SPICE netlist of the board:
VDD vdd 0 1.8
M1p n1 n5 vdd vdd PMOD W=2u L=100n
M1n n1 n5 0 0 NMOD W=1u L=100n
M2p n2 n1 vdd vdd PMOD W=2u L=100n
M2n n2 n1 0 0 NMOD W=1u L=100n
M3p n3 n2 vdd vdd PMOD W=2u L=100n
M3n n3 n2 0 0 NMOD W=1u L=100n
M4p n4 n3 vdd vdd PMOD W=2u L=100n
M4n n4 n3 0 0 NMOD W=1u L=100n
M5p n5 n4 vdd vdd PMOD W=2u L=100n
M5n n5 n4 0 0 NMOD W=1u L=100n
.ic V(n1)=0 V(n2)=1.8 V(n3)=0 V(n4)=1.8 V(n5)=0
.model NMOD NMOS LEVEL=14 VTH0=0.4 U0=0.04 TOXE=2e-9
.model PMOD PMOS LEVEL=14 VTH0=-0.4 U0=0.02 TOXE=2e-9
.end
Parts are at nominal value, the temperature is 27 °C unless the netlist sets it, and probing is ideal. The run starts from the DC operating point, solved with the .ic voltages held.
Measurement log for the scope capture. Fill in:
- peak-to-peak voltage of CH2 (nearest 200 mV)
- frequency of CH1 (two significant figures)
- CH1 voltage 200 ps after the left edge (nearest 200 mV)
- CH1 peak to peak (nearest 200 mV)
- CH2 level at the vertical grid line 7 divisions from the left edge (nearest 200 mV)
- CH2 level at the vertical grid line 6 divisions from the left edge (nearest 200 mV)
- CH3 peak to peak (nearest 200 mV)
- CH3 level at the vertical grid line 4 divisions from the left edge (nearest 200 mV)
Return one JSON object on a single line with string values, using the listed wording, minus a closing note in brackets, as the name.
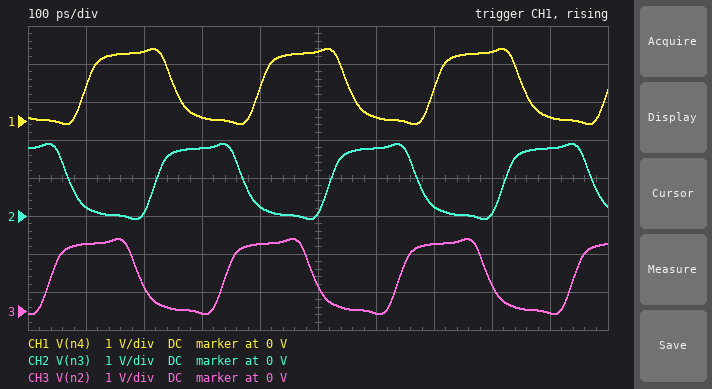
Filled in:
{"peak-to-peak voltage of CH2": "2.0 V", "frequency of CH1": "3.3 GHz", "CH1 voltage 200 ps after the left edge": "1.8 V", "CH1 peak to peak": "2.0 V", "CH2 level at the vertical grid line 7 divisions from the left edge": "200 mV", "CH2 level at the vertical grid line 6 divisions from the left edge": "1.8 V", "CH3 peak to peak": "2.0 V", "CH3 level at the vertical grid line 4 divisions from the left edge": "1.8 V"}
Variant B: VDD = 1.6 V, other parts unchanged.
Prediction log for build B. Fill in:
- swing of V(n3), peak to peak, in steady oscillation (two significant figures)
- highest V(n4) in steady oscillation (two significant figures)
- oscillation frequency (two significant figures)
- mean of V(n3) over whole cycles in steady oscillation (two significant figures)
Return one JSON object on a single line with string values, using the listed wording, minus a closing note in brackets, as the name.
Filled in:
{"swing of V(n3), peak to peak, in steady oscillation": "1.8 V", "highest V(n4) in steady oscillation": "1.7 V", "oscillation frequency": "2.9 GHz", "mean of V(n3) over whole cycles in steady oscillation": "820 mV"}
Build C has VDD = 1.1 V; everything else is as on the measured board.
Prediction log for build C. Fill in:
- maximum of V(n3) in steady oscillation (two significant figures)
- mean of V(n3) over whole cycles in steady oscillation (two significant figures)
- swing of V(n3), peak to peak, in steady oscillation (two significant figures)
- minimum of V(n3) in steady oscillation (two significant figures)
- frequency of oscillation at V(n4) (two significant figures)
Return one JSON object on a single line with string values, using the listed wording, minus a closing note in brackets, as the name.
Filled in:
{"maximum of V(n3) in steady oscillation": "1.2 V", "mean of V(n3) over whole cycles in steady oscillation": "560 mV", "swing of V(n3), peak to peak, in steady oscillation": "1.3 V", "minimum of V(n3) in steady oscillation": "-110 mV", "frequency of oscillation at V(n4)": "1.5 GHz"}
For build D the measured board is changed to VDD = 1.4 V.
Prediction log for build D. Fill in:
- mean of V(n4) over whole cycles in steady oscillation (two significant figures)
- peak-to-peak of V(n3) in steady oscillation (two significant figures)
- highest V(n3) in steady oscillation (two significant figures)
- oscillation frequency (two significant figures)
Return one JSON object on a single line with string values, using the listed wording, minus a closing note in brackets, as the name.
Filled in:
{"mean of V(n4) over whole cycles in steady oscillation": "710 mV", "peak-to-peak of V(n3) in steady oscillation": "1.6 V", "highest V(n3) in steady oscillation": "1.5 V", "oscillation frequency": "2.4 GHz"}
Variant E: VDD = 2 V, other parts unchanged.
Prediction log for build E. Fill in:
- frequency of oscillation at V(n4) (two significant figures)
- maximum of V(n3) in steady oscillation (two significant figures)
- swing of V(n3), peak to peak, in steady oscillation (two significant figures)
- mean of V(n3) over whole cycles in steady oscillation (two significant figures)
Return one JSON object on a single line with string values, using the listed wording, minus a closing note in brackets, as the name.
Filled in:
{"frequency of oscillation at V(n4)": "3.7 GHz", "maximum of V(n3) in steady oscillation": "2.1 V", "swing of V(n3), peak to peak, in steady oscillation": "2.2 V", "mean of V(n3) over whole cycles in steady oscillation": "1.0 V"}
